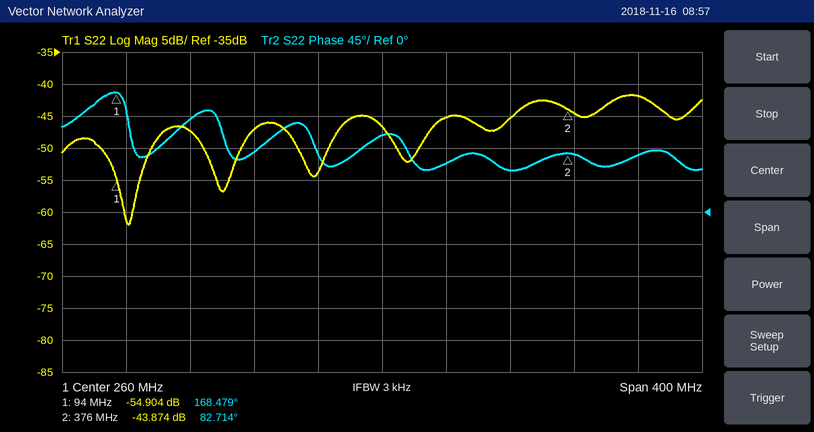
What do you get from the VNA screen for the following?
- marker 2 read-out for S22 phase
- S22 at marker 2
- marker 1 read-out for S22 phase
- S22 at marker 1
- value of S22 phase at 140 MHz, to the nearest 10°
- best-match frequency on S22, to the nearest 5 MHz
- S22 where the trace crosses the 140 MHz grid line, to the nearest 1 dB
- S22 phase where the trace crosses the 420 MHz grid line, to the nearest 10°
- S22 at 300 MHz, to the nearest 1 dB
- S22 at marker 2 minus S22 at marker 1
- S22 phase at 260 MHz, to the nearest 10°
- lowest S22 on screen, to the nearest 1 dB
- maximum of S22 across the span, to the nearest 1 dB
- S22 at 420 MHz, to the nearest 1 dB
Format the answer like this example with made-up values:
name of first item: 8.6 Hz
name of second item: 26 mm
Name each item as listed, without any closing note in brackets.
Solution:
marker 2 read-out for S22 phase: 82.714°
S22 at marker 2: -43.874 dB
marker 1 read-out for S22 phase: 168.479°
S22 at marker 1: -54.904 dB
value of S22 phase at 140 MHz, to the nearest 10°: 130°
best-match frequency on S22, to the nearest 5 MHz: 100 MHz
S22 where the trace crosses the 140 MHz grid line, to the nearest 1 dB: -47 dB
S22 phase where the trace crosses the 420 MHz grid line, to the nearest 10°: 80°
S22 at 300 MHz, to the nearest 1 dB: -45 dB
S22 at marker 2 minus S22 at marker 1: 11.030 dB
S22 phase at 260 MHz, to the nearest 10°: 110°
lowest S22 on screen, to the nearest 1 dB: -62 dB
maximum of S22 across the span, to the nearest 1 dB: -42 dB
S22 at 420 MHz, to the nearest 1 dB: -42 dB
